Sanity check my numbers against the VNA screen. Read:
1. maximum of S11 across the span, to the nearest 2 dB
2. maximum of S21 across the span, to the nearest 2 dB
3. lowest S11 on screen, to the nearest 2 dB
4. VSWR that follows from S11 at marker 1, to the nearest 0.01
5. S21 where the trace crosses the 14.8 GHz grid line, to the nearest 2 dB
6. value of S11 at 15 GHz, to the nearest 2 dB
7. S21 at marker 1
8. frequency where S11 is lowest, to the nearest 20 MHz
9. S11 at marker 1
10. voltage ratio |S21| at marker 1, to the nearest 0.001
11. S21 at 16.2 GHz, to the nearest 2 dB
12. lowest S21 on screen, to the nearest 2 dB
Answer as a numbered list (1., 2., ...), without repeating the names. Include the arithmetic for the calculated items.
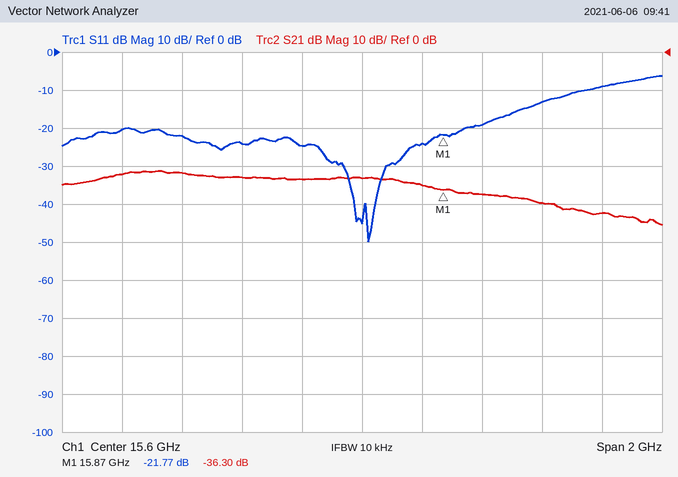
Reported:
1. -6 dB
2. -32 dB
3. -50 dB
4. (1 + 0.0816)/(1 − 0.0816) ≈ 1.18
5. -32 dB
6. -22 dB
7. -36.30 dB
8. 15.62 GHz
9. -21.77 dB
10. 10^(-36.3/20) ≈ 0.015
11. -40 dB
12. -46 dB
